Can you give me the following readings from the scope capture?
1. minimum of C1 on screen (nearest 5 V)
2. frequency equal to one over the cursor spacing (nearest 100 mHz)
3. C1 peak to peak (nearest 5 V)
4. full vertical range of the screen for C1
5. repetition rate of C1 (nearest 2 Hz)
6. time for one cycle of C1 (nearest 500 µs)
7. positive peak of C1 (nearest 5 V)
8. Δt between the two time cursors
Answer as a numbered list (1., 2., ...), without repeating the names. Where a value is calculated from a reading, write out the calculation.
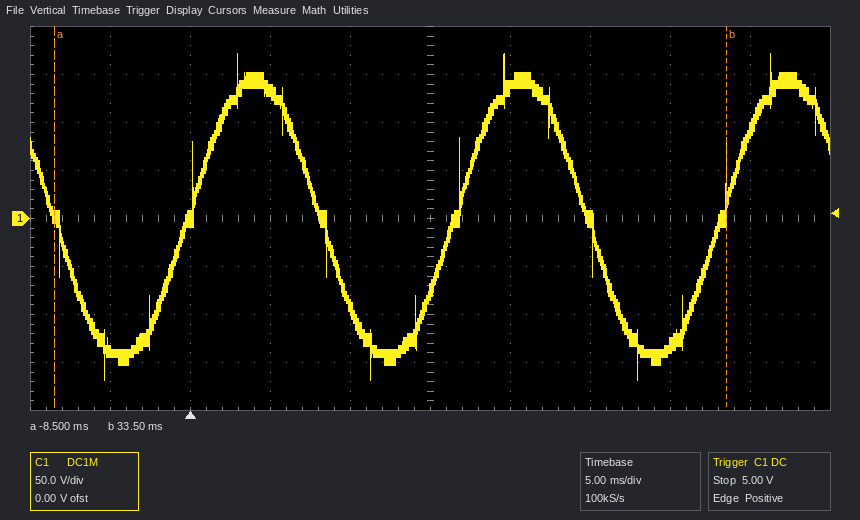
1. -170 V
2. 1 / 42.0 ms ≈ 23.8 Hz
3. 170 V − (-170 V) = 340 V
4. 400 V
5. 1 / 16.5 ms ≈ 60.6 Hz, so 60 Hz to the nearest 2 Hz
6. 16.5 ms
7. 170 V
8. 33.5 ms − (-8.5 ms) = 42.0 ms
